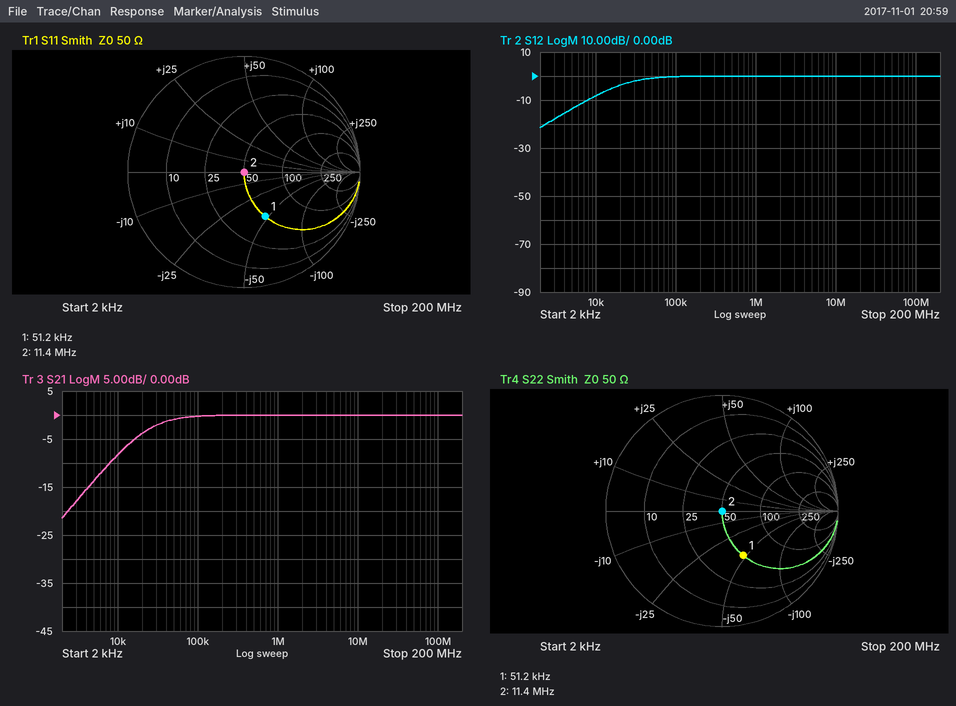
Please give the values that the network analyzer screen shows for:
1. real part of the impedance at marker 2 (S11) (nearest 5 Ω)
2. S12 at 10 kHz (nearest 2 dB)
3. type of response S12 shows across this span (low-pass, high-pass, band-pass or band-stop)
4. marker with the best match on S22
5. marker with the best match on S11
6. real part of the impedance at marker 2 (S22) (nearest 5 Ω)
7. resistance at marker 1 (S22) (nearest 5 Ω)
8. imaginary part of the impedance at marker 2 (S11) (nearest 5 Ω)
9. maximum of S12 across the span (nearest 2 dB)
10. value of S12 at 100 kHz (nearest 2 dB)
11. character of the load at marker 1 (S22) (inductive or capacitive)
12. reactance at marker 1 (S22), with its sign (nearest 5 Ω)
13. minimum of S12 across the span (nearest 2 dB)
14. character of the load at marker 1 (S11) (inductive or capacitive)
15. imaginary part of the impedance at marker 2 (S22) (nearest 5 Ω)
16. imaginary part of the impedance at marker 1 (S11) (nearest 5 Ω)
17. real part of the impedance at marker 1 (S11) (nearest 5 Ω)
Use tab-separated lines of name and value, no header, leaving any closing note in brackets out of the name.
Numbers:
real part of the impedance at marker 2 (S11)	50 Ω
S12 at 10 kHz	-8 dB
type of response S12 shows across this span	high-pass
marker with the best match on S22	marker 2
marker with the best match on S11	marker 2
real part of the impedance at marker 2 (S22)	50 Ω
resistance at marker 1 (S22)	50 Ω
imaginary part of the impedance at marker 2 (S11)	0 Ω
maximum of S12 across the span	0 dB
value of S12 at 100 kHz	0 dB
character of the load at marker 1 (S22)	capacitive
reactance at marker 1 (S22), with its sign	-45 Ω
minimum of S12 across the span	-22 dB
character of the load at marker 1 (S11)	capacitive
imaginary part of the impedance at marker 2 (S22)	0 Ω
imaginary part of the impedance at marker 1 (S11)	-45 Ω
real part of the impedance at marker 1 (S11)	50 Ω
